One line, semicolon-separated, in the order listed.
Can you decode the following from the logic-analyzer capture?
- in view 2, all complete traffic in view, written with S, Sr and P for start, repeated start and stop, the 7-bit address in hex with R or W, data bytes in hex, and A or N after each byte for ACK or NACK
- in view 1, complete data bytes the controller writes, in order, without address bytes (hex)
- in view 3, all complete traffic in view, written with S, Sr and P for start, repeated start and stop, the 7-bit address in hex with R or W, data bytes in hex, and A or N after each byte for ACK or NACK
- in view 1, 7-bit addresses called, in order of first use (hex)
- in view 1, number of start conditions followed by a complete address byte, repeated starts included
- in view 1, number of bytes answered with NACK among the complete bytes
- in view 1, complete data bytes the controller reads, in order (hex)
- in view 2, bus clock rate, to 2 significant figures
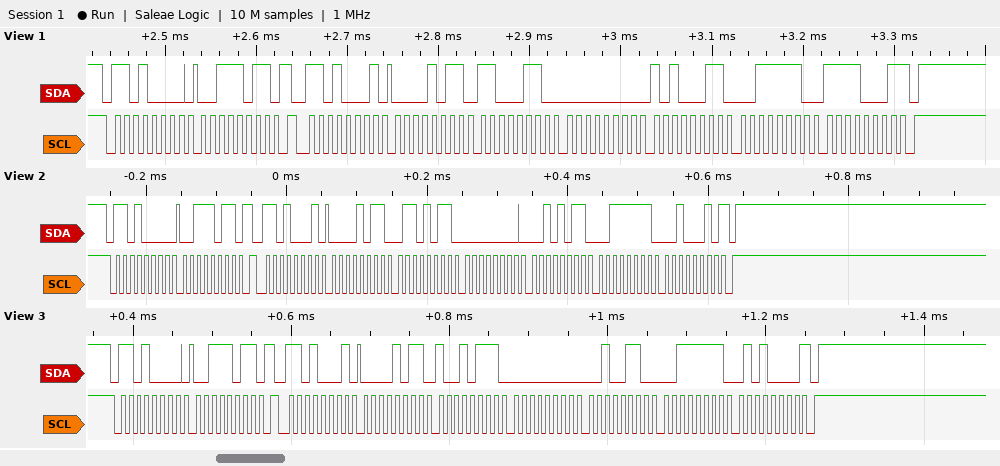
S 68W A 3B A Sr 68R A 0B A 6B A 00 A 2B A 3F A 22 N P; 3B; S 68W A 3B A Sr 68R A 0B A 97 A 00 A 26 A 3F A 50 N P; 0x68; 2; 1; 0B C6 00 A3 3E F1; 100 kHz
